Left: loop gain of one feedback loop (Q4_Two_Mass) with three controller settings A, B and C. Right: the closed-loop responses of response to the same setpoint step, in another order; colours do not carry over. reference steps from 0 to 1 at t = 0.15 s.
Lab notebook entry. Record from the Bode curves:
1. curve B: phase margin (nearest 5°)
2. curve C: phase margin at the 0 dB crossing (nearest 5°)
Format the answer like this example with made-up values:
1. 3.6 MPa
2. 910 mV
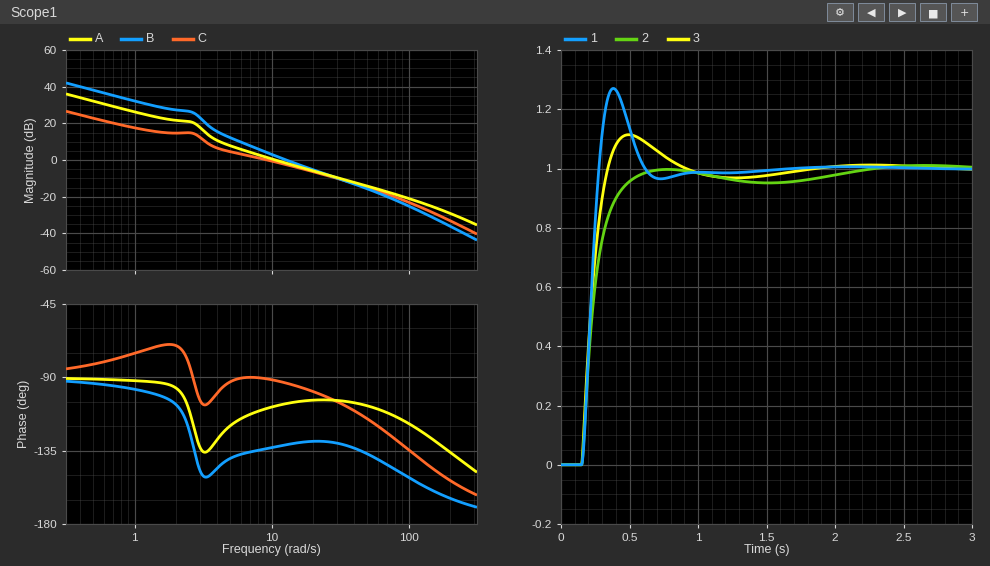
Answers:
1. 50°
2. 90°
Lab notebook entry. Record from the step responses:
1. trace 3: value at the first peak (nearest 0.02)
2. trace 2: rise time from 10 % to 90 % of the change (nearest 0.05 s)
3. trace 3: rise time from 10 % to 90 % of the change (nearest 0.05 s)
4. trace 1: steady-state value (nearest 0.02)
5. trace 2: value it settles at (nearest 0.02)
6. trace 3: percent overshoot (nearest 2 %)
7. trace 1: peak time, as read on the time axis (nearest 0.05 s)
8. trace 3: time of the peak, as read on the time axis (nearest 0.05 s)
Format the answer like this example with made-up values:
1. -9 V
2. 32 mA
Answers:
1. 1.12
2. 0.25 s
3. 0.15 s
4. 1.00
5. 1.00
6. 12 %
7. 0.40 s
8. 0.50 s
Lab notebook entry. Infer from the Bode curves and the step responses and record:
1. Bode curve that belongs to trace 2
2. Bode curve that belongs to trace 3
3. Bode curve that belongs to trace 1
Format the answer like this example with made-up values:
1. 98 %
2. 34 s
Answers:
1. C
2. A
3. B
